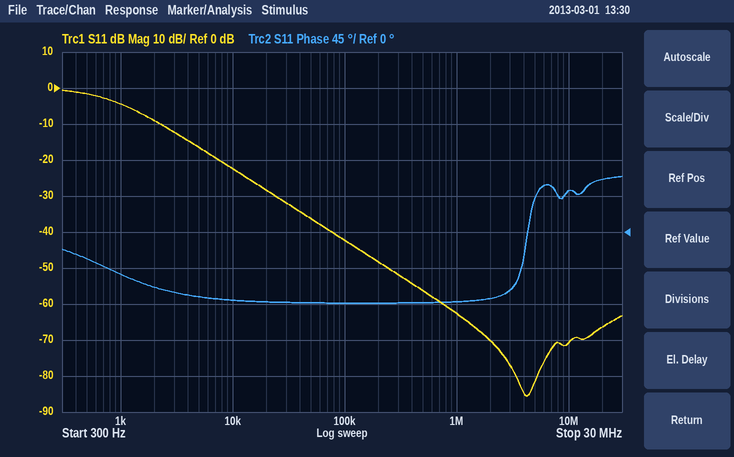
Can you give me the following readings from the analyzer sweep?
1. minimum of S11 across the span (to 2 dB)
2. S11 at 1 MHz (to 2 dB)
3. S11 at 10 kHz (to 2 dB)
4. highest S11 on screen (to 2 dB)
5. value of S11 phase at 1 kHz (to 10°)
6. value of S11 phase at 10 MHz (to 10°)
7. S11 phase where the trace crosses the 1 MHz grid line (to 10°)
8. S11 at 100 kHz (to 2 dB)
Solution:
-86 dB
-62 dB
-22 dB
0 dB
-50°
50°
-90°
-42 dB
